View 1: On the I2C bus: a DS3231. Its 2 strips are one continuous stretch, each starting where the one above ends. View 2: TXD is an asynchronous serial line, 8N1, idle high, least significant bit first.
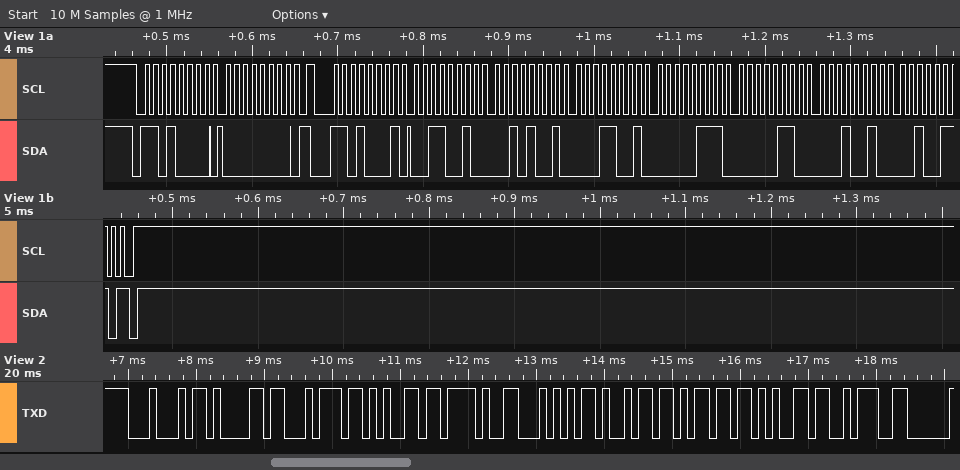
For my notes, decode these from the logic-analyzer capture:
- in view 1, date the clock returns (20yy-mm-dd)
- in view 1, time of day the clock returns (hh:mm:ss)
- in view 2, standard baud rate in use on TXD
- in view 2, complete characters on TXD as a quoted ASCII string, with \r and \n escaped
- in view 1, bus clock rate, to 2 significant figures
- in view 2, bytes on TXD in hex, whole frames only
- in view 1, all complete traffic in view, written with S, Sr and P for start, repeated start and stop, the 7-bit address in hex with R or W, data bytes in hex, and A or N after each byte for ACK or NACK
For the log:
2026-12-06
19:29:32
9600 baud
"Date/Time:"
100 kHz
44 61 74 65 2F 54 69 6D 65 3A
S 68W A 00 A Sr 68R A 32 A 29 A 19 A 07 A 06 A 12 A 26 N P
